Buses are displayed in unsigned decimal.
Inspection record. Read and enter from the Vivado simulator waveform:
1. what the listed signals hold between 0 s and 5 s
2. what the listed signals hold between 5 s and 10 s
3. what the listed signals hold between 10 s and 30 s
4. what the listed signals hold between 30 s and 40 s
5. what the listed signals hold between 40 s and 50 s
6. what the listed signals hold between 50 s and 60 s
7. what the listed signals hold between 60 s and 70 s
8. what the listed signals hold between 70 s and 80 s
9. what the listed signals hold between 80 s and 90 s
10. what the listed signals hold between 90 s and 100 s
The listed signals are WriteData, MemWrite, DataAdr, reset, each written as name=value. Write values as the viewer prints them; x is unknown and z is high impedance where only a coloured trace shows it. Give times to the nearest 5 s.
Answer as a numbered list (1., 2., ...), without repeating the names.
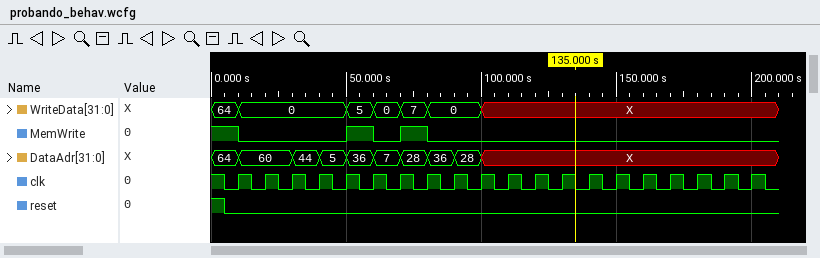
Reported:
1. WriteData=64, MemWrite=1, DataAdr=64, reset=1
2. WriteData=64, MemWrite=1, DataAdr=64, reset=0
3. WriteData=0, MemWrite=0, DataAdr=60, reset=0
4. WriteData=0, MemWrite=0, DataAdr=44, reset=0
5. WriteData=0, MemWrite=0, DataAdr=5, reset=0
6. WriteData=5, MemWrite=1, DataAdr=36, reset=0
7. WriteData=0, MemWrite=0, DataAdr=7, reset=0
8. WriteData=7, MemWrite=1, DataAdr=28, reset=0
9. WriteData=0, MemWrite=0, DataAdr=36, reset=0
10. WriteData=0, MemWrite=0, DataAdr=28, reset=0
